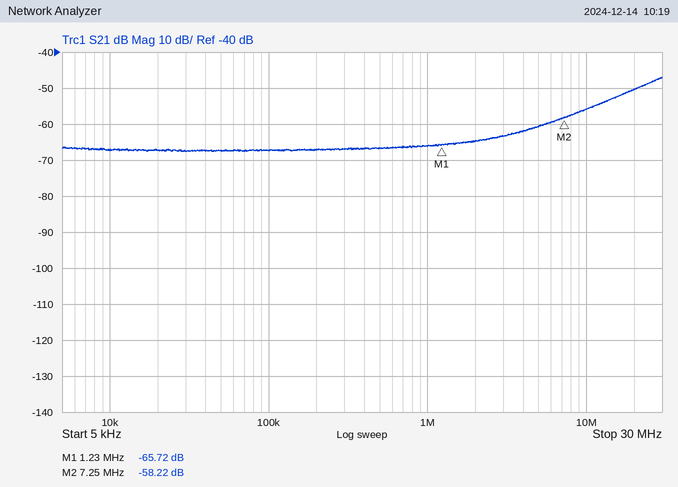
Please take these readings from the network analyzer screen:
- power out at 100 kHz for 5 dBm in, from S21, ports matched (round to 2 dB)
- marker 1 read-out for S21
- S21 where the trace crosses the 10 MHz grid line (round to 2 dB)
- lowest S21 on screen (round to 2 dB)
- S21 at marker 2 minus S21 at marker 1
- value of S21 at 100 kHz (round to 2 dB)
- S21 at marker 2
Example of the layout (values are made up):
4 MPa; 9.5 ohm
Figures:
-62 dBm; -65.72 dB; -56 dB; -68 dB; 7.50 dB; -68 dB; -58.22 dB
